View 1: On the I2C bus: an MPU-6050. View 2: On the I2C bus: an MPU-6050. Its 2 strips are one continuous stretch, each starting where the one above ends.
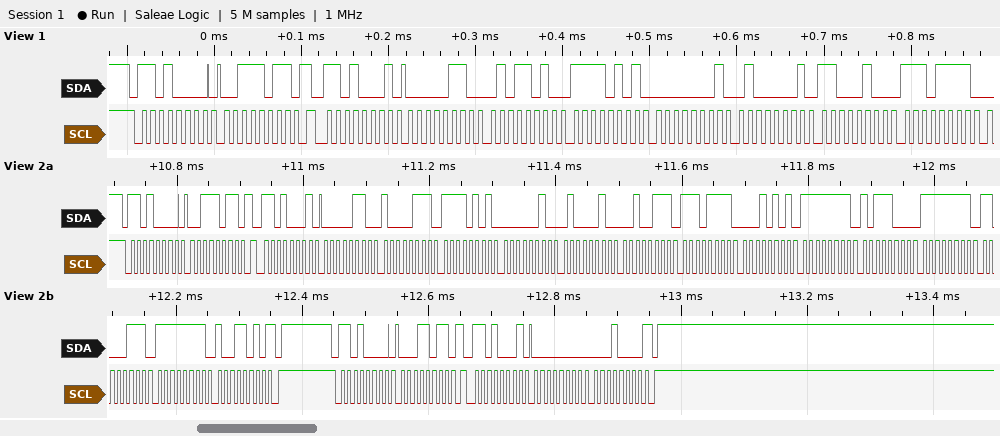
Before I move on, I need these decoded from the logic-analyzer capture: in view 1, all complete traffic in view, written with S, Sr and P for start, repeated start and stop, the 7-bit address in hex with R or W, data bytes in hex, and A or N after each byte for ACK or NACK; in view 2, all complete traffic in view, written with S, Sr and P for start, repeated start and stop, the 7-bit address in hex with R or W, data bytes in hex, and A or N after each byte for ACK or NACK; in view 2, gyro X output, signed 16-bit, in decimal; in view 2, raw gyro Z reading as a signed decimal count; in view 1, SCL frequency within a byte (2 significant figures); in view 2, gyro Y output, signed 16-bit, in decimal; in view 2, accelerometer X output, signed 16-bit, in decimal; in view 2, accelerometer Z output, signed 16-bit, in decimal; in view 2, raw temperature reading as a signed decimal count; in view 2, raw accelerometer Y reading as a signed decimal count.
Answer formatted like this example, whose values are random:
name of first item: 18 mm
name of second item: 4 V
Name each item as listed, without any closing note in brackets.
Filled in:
in view 1, all complete traffic in view, written with S, Sr and P for start, repeated start and stop, the 7-bit address in hex with R or W, data bytes in hex, and A or N after each byte for ACK or NACK: S 68W A 3B A Sr 68R A 06 A 5A A F5 A 01 A 41 A C4 A EF A
in view 2, all complete traffic in view, written with S, Sr and P for start, repeated start and stop, the 7-bit address in hex with R or W, data bytes in hex, and A or N after each byte for ACK or NACK: S 68W A 3B A Sr 68R A 06 A 87 A F5 A 02 A 42 A 27 A EF A 15 A FF A B8 A FF A C7 A FF A 9A N P S 68W A 1B A Sr 68R A 00 A 10 N P
in view 2, gyro X output, signed 16-bit, in decimal: -72
in view 2, raw gyro Z reading as a signed decimal count: -102
in view 1, SCL frequency within a byte: 100 kHz
in view 2, gyro Y output, signed 16-bit, in decimal: -57
in view 2, accelerometer X output, signed 16-bit, in decimal: 1671
in view 2, accelerometer Z output, signed 16-bit, in decimal: 16935
in view 2, raw temperature reading as a signed decimal count: -4331
in view 2, raw accelerometer Y reading as a signed decimal count: -2814
